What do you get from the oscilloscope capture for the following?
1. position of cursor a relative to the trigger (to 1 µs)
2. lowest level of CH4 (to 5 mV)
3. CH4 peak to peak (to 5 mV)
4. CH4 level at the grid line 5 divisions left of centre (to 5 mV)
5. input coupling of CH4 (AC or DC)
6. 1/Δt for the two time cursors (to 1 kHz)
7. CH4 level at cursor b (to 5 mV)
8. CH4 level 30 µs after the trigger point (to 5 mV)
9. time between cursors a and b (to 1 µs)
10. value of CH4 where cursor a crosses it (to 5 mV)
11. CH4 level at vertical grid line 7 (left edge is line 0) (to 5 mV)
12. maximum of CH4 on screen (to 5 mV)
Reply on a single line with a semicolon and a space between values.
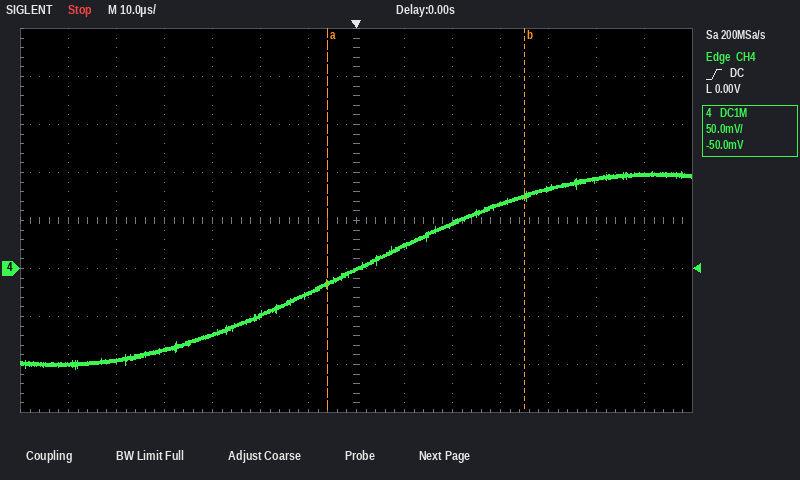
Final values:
-6 µs; -105 mV; 205 mV; -95 mV; DC; 24 kHz; 75 mV; 65 mV; 41 µs; -15 mV; 0 mV; 100 mV
